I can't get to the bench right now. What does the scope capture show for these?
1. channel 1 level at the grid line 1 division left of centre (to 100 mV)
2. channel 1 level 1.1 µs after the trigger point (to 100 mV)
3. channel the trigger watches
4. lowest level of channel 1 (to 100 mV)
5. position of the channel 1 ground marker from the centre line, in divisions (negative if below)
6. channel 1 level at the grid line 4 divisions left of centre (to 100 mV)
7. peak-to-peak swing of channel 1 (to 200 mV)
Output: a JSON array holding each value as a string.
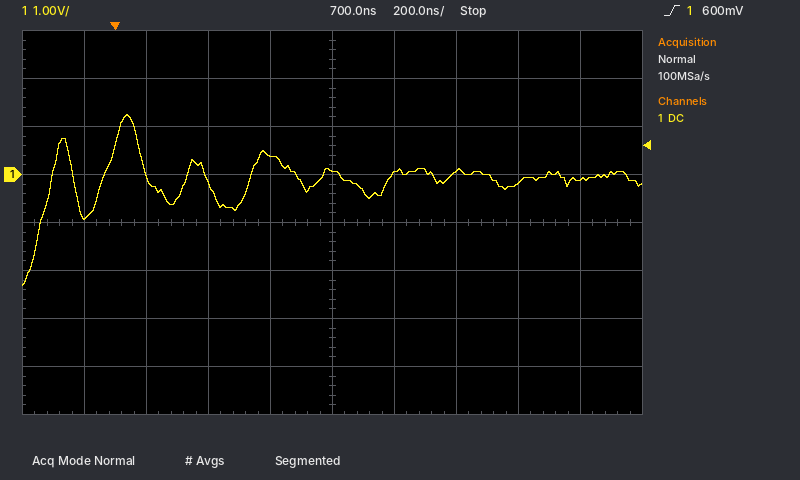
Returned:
["400 mV", "100 mV", "channel 1", "-2.3 V", "+1.0 div", "-900 mV", "3.6 V"]
